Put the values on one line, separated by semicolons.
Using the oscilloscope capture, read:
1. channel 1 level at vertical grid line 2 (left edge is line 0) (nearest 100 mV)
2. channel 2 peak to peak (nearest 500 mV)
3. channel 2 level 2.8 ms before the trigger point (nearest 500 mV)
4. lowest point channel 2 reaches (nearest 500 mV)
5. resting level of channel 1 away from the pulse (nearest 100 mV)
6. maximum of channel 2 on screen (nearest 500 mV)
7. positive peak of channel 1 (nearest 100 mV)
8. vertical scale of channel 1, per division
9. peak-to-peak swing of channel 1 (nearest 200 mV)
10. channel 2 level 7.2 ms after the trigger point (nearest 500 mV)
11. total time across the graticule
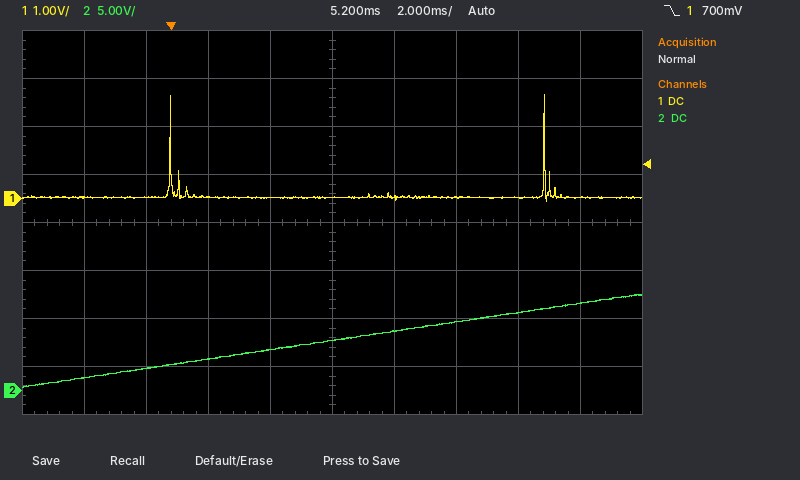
0.0 V; 9.5 V; 1.5 V; 500 mV; 0.0 V; 10.0 V; 2.2 V; 1 V; 2.2 V; 6.0 V; 20 ms
